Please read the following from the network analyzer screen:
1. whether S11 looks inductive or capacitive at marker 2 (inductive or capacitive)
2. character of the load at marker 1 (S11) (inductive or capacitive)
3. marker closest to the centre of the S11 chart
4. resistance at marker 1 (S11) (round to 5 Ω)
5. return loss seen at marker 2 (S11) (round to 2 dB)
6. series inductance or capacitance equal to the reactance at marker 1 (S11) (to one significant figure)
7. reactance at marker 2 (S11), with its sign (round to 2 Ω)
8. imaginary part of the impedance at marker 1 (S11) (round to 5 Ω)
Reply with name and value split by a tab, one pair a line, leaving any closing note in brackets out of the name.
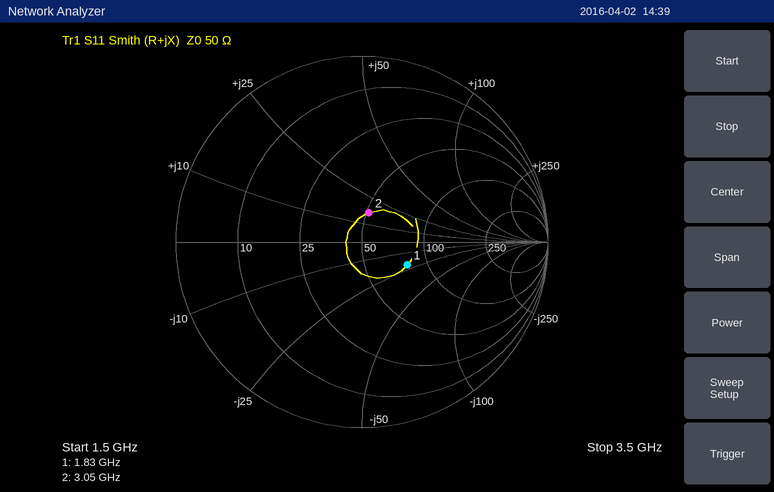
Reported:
whether S11 looks inductive or capacitive at marker 2	inductive
character of the load at marker 1 (S11)	capacitive
marker closest to the centre of the S11 chart	marker 2
resistance at marker 1 (S11)	80 Ω
return loss seen at marker 2 (S11)	16 dB
series inductance or capacitance equal to the reactance at marker 1 (S11)	4 pF
reactance at marker 2 (S11), with its sign	+16 Ω
imaginary part of the impedance at marker 1 (S11)	-20 Ω
